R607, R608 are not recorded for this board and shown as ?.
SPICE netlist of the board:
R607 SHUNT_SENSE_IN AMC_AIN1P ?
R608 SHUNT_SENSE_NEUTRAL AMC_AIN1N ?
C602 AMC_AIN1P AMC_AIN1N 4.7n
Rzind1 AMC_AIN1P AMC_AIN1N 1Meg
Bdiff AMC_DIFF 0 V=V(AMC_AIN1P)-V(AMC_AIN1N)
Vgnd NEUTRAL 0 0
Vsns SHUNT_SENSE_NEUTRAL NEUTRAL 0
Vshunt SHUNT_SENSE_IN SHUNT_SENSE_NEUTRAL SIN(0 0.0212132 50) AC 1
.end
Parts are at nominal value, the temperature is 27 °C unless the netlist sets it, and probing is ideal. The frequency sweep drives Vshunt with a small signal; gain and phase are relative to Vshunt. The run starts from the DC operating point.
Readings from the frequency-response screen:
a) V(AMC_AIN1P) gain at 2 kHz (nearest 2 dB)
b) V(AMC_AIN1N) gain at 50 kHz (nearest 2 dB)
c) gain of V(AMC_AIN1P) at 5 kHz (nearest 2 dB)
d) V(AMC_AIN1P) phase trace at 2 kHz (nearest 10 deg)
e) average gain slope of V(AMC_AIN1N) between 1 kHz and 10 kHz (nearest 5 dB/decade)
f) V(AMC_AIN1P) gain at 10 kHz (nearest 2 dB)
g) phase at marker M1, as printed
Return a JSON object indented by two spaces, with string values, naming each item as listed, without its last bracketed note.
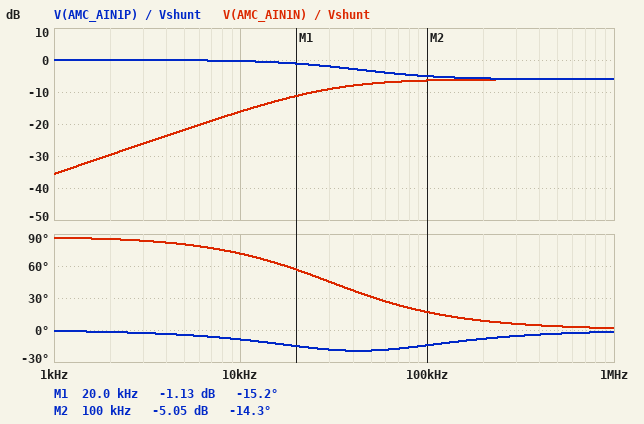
{
  "V(AMC_AIN1P) gain at 2 kHz": "0 dB",
  "V(AMC_AIN1N) gain at 50 kHz": "-8 dB",
  "gain of V(AMC_AIN1P) at 5 kHz": "0 dB",
  "V(AMC_AIN1P) phase trace at 2 kHz": "0 deg",
  "average gain slope of V(AMC_AIN1N) between 1 kHz and 10 kHz": "20 dB/decade",
  "V(AMC_AIN1P) gain at 10 kHz": "0 dB",
  "phase at marker M1, as printed": "-15.2 deg"
}
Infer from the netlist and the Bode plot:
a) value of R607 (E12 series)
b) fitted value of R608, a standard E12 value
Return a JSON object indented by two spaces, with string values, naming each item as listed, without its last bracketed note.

{
  "value of R607": "560 Ω",
  "fitted value of R608, a standard E12 value": "560 Ω"
}
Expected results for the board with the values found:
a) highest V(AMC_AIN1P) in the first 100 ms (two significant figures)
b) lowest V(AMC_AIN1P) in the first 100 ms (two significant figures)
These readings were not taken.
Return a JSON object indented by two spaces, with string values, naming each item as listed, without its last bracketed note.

{
  "highest V(AMC_AIN1P) in the first 100 ms": "21 mV",
  "lowest V(AMC_AIN1P) in the first 100 ms": "-21 mV"
}
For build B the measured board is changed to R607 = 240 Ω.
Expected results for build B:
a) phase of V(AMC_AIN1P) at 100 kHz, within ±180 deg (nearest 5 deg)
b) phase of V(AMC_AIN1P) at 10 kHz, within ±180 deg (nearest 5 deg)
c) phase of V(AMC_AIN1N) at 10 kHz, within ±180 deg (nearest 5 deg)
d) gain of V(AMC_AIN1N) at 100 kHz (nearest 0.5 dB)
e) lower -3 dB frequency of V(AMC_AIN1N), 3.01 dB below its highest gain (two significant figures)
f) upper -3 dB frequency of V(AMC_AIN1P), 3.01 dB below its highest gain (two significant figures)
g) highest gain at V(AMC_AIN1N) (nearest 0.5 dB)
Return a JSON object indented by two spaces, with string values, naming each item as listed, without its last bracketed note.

{
  "phase of V(AMC_AIN1P) at 100 kHz, within ±180 deg": "-10 deg",
  "phase of V(AMC_AIN1P) at 10 kHz, within ±180 deg": "-5 deg",
  "phase of V(AMC_AIN1N) at 10 kHz, within ±180 deg": "75 deg",
  "gain of V(AMC_AIN1N) at 100 kHz": "-4.0 dB",
  "lower -3 dB frequency of V(AMC_AIN1N), 3.01 dB below its highest gain": "42 kHz",
  "upper -3 dB frequency of V(AMC_AIN1P), 3.01 dB below its highest gain": "300 kHz",
  "highest gain at V(AMC_AIN1N)": "-3.0 dB"
}
